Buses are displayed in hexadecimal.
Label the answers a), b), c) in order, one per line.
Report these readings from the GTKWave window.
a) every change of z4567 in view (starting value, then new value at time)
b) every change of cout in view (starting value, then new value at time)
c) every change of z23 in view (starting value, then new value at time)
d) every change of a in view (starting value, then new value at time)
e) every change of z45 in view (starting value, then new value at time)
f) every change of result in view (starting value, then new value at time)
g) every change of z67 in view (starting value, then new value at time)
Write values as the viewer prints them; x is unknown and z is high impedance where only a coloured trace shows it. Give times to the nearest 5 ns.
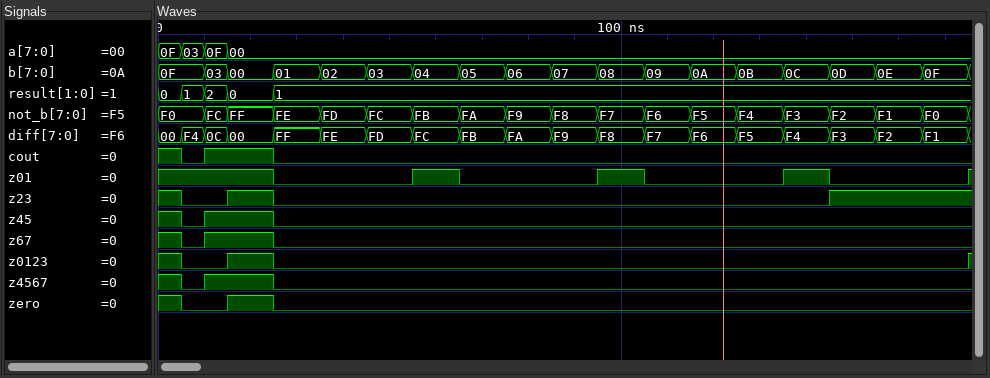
a) 1, 0 at 5 ns, 1 at 10 ns, 0 at 25 ns
b) 1, 0 at 5 ns, 1 at 10 ns, 0 at 25 ns
c) 1, 0 at 5 ns, 1 at 15 ns, 0 at 25 ns, 1 at 145 ns
d) 0F, 03 at 5 ns, 0F at 10 ns, 00 at 15 ns
e) 1, 0 at 5 ns, 1 at 10 ns, 0 at 25 ns
f) 0, 1 at 5 ns, 2 at 10 ns, 0 at 15 ns, 1 at 25 ns
g) 1, 0 at 5 ns, 1 at 10 ns, 0 at 25 ns
